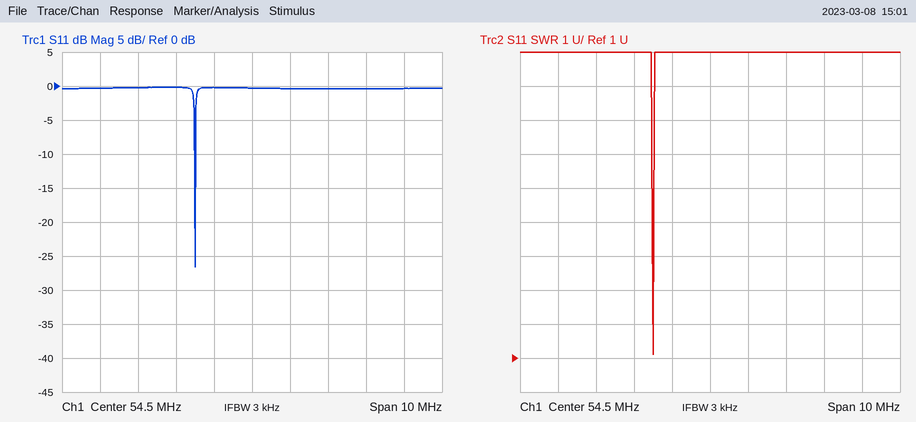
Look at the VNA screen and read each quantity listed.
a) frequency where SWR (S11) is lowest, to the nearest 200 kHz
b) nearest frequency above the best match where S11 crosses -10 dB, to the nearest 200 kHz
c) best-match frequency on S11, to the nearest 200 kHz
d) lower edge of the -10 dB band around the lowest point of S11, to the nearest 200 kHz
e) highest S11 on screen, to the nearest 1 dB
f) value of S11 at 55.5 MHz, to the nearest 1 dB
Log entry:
53.0 MHz
53.0 MHz
53.0 MHz
53.0 MHz
0 dB
0 dB
